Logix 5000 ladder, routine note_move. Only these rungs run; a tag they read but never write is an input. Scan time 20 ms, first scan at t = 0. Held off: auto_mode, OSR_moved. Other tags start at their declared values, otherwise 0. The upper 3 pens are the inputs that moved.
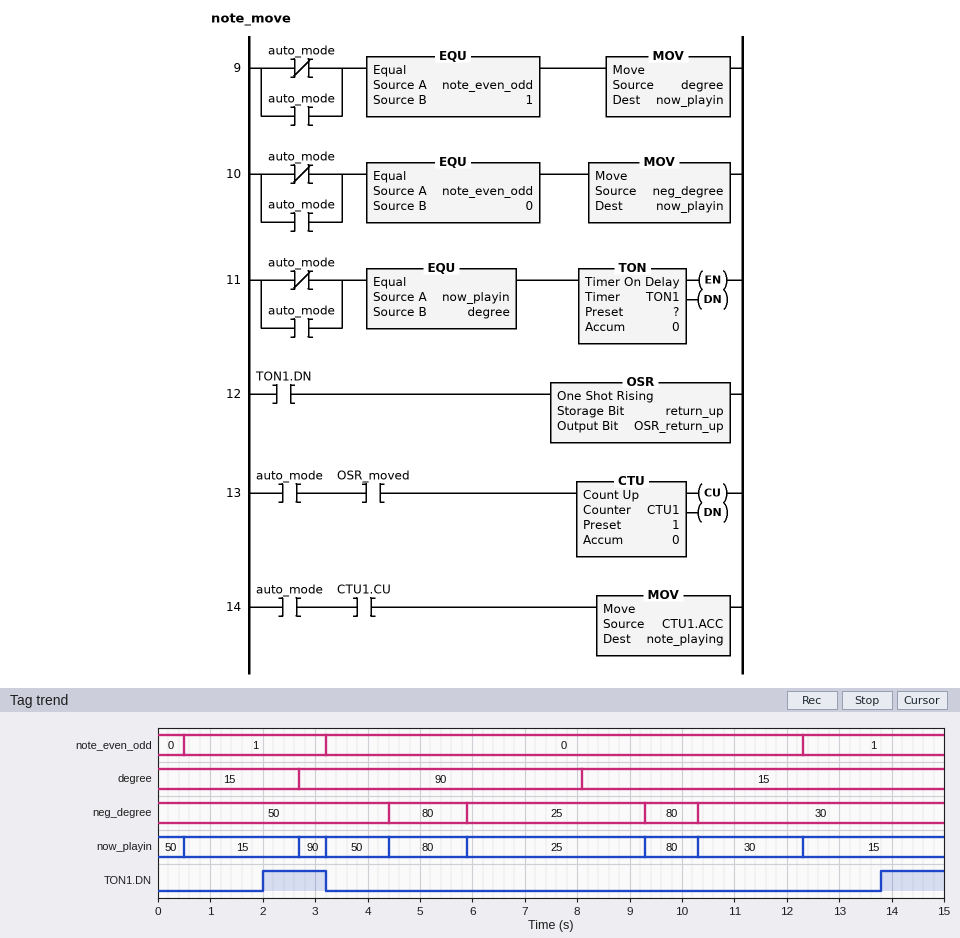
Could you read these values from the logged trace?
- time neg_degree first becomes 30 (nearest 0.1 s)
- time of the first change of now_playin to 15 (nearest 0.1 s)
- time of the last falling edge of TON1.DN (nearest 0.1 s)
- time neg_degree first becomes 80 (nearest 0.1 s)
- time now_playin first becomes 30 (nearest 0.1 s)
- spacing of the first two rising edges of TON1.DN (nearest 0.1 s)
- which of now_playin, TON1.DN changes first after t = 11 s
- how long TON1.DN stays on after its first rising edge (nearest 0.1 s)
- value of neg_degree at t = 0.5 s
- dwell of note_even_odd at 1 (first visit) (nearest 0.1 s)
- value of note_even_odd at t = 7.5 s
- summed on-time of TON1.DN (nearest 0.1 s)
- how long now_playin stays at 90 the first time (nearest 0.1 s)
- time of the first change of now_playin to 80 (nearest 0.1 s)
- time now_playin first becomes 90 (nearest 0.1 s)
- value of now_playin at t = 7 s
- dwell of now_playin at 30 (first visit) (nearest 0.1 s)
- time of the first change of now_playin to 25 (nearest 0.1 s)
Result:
10.3 s
0.5 s
3.2 s
4.4 s
10.3 s
11.8 s
now_playin
1.2 s
50
2.7 s
0
2.4 s
0.5 s
4.4 s
2.7 s
25
2.0 s
5.9 s
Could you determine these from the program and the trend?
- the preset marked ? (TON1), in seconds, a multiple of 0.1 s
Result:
1.5 s
